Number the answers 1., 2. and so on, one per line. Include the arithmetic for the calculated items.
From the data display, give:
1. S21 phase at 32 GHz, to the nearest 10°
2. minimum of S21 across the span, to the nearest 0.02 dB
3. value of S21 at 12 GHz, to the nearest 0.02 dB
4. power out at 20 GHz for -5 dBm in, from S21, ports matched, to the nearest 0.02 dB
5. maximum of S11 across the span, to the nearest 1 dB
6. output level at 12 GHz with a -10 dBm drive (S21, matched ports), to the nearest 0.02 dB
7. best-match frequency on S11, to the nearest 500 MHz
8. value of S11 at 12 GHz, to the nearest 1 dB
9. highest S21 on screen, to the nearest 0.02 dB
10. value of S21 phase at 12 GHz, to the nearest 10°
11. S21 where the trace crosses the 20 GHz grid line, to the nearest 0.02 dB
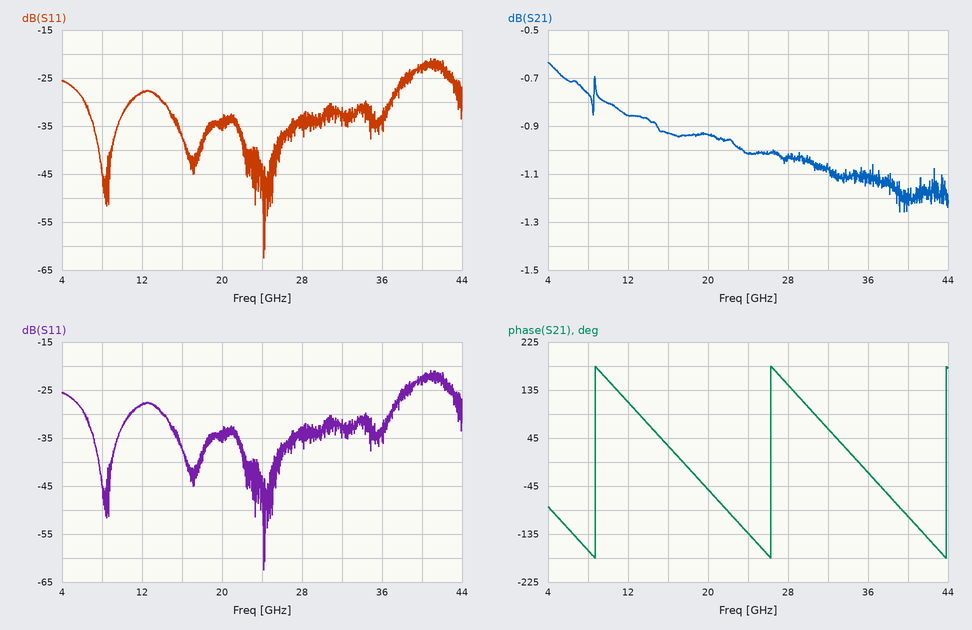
1. 60°
2. -1.26 dB
3. -0.86 dB
4. -5 dBm + (-0.94 dB) = -5.94 dBm
5. -21 dB
6. -10 dBm + (-0.86 dB) = -10.86 dBm
7. 24.0 GHz
8. -28 dB
9. -0.64 dB
10. 110°
11. -0.94 dB
